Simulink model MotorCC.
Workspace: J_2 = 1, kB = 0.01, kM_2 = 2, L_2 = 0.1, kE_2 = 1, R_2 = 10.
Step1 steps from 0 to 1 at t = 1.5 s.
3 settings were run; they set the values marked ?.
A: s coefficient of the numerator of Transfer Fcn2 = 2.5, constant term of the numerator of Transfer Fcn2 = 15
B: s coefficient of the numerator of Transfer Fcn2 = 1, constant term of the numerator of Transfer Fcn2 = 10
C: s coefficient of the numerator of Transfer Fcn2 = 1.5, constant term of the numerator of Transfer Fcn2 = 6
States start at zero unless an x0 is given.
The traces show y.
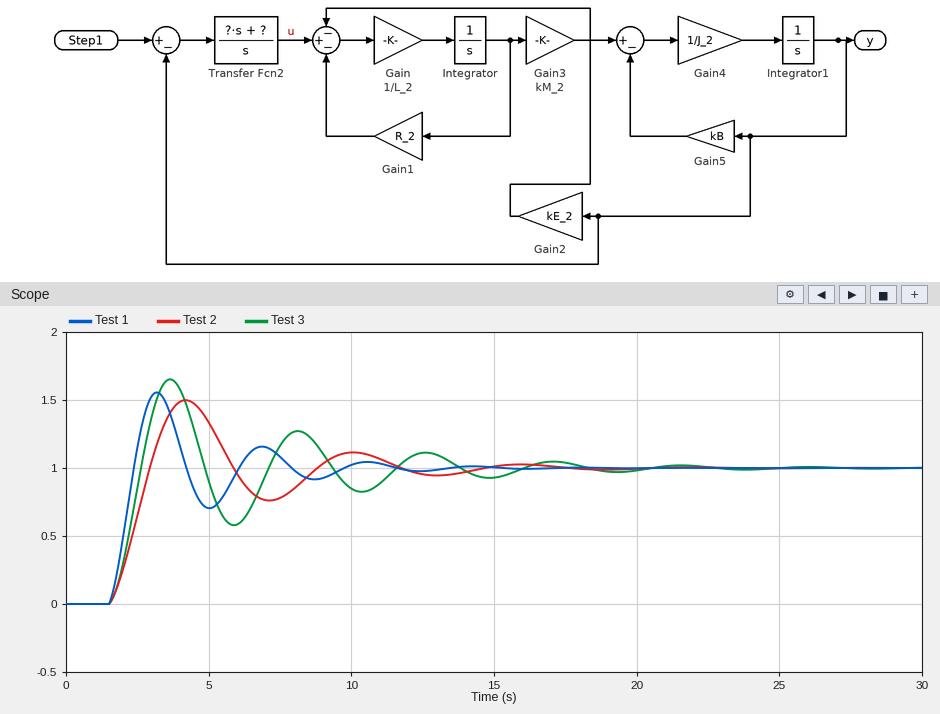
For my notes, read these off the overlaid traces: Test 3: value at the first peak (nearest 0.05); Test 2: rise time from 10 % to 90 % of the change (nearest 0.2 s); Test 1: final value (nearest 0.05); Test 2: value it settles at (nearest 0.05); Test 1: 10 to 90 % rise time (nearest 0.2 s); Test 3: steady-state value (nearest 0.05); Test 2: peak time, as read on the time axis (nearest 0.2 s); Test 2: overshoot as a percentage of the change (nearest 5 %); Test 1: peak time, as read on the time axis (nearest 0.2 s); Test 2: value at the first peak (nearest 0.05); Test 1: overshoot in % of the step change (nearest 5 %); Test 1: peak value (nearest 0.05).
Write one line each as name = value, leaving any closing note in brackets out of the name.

Test 3: value at the first peak = 1.65
Test 2: rise time from 10 % to 90 % of the change = 1.0 s
Test 1: final value = 1.00
Test 2: value it settles at = 1.00
Test 1: 10 to 90 % rise time = 0.6 s
Test 3: steady-state value = 1.00
Test 2: peak time, as read on the time axis = 4.2 s
Test 2: overshoot as a percentage of the change = 50 %
Test 1: peak time, as read on the time axis = 3.2 s
Test 2: value at the first peak = 1.50
Test 1: overshoot in % of the step change = 55 %
Test 1: peak value = 1.55
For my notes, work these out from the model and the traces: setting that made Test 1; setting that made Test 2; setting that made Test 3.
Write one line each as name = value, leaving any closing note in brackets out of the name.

setting that made Test 1 = A
setting that made Test 2 = C
setting that made Test 3 = B
